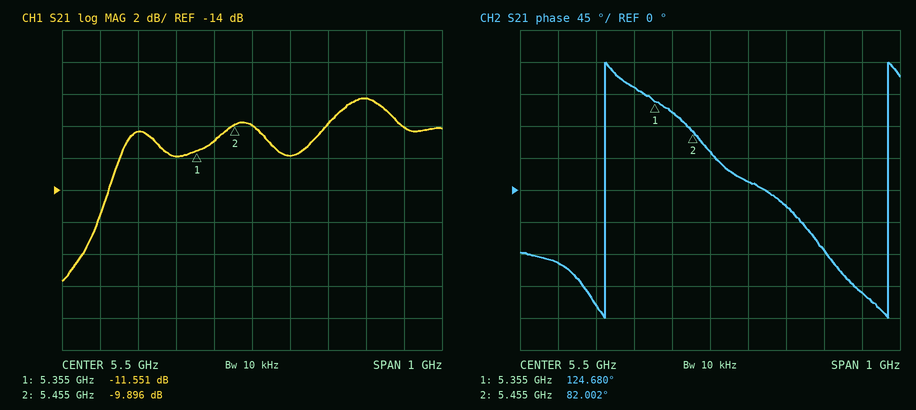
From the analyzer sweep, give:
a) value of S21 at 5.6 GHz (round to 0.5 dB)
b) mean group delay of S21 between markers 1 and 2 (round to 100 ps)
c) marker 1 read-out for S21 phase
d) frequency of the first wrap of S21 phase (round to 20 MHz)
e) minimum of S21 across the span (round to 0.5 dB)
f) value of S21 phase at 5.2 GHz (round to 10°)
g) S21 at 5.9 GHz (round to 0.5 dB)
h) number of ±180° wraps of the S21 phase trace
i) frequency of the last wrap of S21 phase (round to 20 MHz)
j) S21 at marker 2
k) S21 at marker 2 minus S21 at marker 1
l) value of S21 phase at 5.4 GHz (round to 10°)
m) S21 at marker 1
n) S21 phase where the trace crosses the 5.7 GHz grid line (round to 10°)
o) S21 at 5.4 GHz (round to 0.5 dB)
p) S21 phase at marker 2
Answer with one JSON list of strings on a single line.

["-12.0 dB", "1.2 ns", "124.680°", "5.22 GHz", "-19.5 dB", "-160°", "-10.0 dB", "2", "5.96 GHz", "-9.896 dB", "1.655 dB", "110°", "-11.551 dB", "-20°", "-11.0 dB", "82.002°"]
